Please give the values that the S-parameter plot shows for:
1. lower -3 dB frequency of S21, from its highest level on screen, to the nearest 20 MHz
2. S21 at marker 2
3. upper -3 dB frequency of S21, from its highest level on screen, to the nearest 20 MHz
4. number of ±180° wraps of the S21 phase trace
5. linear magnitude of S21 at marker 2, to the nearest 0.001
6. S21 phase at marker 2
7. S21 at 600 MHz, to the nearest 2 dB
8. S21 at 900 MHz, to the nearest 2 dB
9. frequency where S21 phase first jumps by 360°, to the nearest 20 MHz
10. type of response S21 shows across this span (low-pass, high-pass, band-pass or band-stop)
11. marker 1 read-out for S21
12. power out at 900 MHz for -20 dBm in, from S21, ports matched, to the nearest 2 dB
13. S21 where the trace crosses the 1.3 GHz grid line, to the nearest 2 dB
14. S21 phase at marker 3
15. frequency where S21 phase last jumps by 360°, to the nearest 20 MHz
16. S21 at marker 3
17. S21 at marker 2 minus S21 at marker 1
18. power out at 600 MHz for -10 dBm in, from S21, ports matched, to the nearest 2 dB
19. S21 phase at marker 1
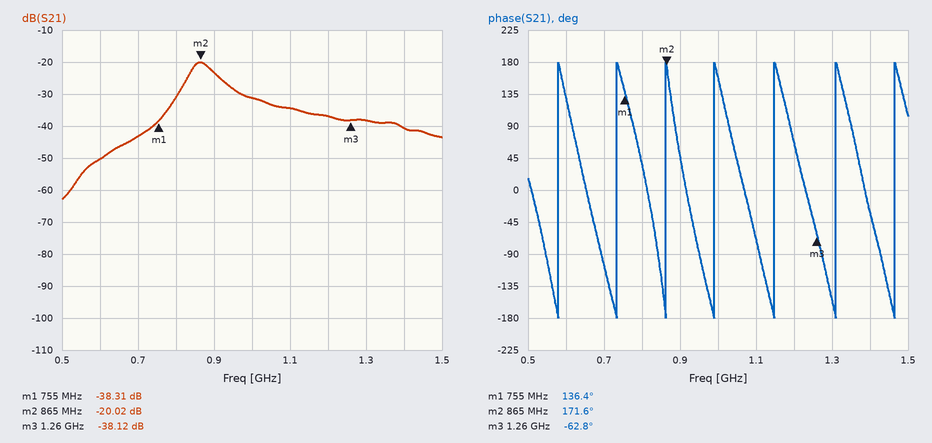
840 MHz
-20.02 dB
900 MHz
7
0.100
171.6°
-50 dB
-24 dB
580 MHz
band-pass
-38.31 dB
-44 dBm
-38 dB
-62.8°
1.46 GHz
-38.12 dB
18.29 dB
-60 dBm
136.4°
